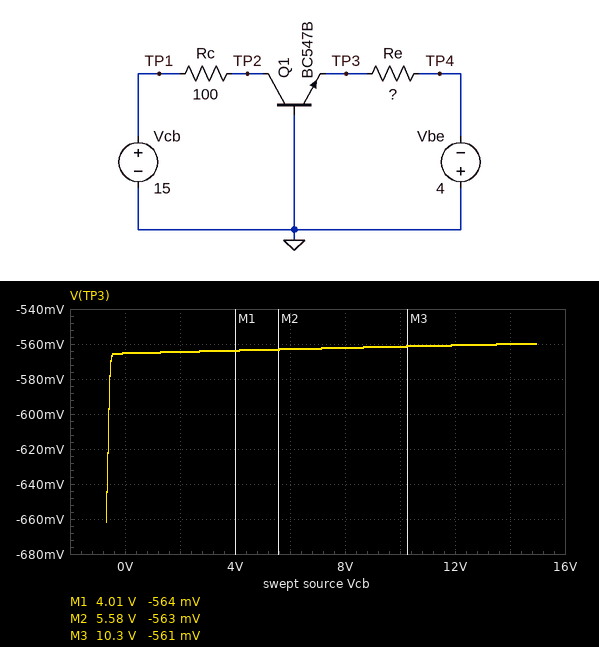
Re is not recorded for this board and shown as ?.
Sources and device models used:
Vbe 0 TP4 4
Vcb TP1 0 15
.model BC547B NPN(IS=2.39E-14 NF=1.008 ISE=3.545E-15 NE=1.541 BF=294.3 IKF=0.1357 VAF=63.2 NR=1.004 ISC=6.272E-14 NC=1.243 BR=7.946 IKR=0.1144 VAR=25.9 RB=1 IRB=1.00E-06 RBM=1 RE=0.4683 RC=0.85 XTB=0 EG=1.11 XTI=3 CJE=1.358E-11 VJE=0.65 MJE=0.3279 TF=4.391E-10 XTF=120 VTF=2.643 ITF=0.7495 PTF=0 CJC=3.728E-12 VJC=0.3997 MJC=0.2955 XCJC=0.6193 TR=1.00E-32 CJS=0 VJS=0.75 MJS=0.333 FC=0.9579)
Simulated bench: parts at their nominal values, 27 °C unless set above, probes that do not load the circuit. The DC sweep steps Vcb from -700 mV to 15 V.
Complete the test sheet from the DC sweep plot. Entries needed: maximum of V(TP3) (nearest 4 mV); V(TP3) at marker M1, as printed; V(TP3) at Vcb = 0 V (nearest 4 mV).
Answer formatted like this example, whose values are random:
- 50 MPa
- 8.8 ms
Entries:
- -560 mV
- -564 mV
- -564 mV
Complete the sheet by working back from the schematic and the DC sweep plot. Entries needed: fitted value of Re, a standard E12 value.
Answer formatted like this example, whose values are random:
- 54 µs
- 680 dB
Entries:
- 56 kΩ
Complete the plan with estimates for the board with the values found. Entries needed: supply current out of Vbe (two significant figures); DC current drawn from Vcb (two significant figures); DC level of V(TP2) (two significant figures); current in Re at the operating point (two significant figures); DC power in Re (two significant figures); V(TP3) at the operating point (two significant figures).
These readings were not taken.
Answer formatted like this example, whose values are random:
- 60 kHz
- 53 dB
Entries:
- 61 µA
- 61 µA
- 15 V
- 61 µA
- 210 µW
- -560 mV
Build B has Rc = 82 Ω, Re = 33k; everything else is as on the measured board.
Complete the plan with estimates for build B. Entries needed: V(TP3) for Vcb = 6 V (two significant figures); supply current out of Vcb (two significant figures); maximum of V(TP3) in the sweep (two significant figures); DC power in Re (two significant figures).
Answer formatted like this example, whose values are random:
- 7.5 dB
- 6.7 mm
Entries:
- -580 mV
- 100 µA
- -570 mV
- 360 µW
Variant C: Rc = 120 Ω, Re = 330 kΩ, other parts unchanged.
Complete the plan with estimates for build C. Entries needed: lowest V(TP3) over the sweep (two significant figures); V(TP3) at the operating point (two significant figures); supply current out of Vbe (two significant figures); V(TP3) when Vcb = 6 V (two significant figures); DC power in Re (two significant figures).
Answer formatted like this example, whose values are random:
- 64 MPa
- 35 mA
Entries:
- -660 mV
- -510 mV
- 11 µA
- -520 mV
- 37 µW
